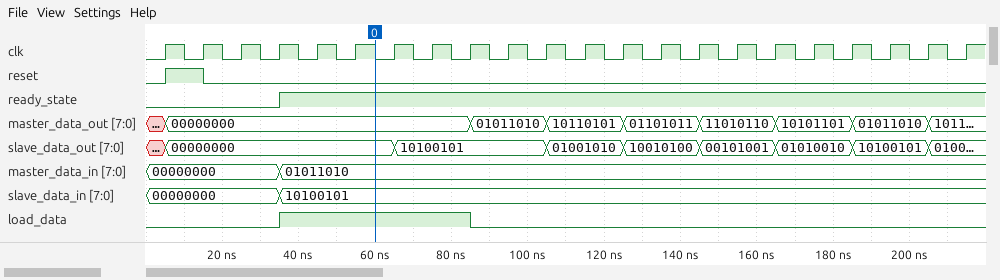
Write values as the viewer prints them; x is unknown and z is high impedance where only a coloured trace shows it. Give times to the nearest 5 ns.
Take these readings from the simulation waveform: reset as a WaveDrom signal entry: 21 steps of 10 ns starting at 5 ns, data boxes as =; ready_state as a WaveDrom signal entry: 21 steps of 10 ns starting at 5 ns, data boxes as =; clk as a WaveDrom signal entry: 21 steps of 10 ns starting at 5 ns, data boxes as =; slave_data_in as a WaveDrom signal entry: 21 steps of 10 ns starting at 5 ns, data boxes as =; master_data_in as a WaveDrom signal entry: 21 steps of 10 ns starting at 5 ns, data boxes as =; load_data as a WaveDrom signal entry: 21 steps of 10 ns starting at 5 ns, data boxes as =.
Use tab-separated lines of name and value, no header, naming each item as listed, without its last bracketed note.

reset as a WaveDrom signal entry: 21 steps of 10 ns starting at 5 ns, data boxes as =	{name: 'reset', wave: '10...................'}
ready_state as a WaveDrom signal entry: 21 steps of 10 ns starting at 5 ns, data boxes as =	{name: 'ready_state', wave: '0..1.................'}
clk as a WaveDrom signal entry: 21 steps of 10 ns starting at 5 ns, data boxes as =	{name: 'clk', wave: 'p....................'}
slave_data_in as a WaveDrom signal entry: 21 steps of 10 ns starting at 5 ns, data boxes as =	{name: 'slave_data_in', wave: '=..=.................', data: '00000000 10100101'}
master_data_in as a WaveDrom signal entry: 21 steps of 10 ns starting at 5 ns, data boxes as =	{name: 'master_data_in', wave: '=..=.................', data: '00000000 01011010'}
load_data as a WaveDrom signal entry: 21 steps of 10 ns starting at 5 ns, data boxes as =	{name: 'load_data', wave: '0..1....0............'}
